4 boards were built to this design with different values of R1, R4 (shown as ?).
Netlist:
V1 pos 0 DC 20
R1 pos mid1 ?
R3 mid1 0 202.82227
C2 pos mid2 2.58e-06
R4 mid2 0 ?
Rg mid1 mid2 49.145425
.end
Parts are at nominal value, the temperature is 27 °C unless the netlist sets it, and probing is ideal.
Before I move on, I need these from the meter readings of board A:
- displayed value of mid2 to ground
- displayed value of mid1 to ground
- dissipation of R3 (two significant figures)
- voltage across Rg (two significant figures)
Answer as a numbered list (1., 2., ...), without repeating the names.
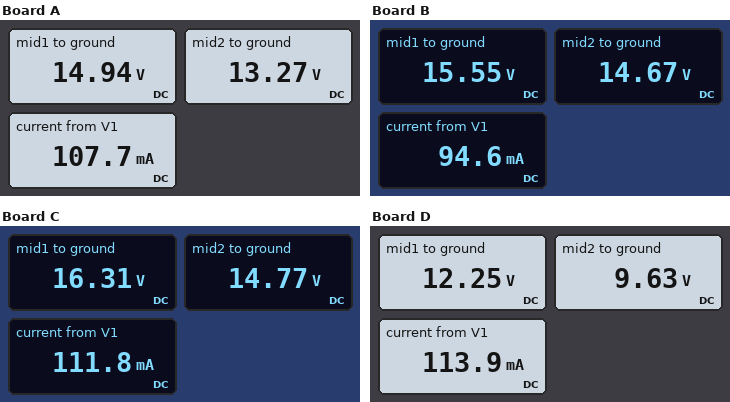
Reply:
1. 13.27 V
2. 14.94 V
3. 1.1 W
4. 1.7 V
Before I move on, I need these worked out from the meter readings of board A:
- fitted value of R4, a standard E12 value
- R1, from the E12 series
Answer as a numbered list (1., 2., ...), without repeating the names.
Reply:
1. 390 Ω
2. 47 Ω
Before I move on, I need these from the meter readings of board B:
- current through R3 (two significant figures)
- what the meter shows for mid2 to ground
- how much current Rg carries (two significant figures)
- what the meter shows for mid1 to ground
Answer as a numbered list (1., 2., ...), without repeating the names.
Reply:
1. 77 mA
2. 14.67 V
3. 18 mA
4. 15.55 V
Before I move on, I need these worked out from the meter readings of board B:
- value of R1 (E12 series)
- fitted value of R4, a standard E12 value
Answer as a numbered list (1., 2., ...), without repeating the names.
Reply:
1. 47 Ω
2. 820 Ω
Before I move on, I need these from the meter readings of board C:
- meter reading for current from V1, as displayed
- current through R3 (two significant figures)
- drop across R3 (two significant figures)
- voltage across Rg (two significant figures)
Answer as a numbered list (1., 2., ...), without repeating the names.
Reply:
1. 111.8 mA
2. 80 mA
3. 16 V
4. 1.5 V
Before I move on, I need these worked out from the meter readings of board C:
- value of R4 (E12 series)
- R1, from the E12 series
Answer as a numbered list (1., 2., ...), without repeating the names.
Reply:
1. 470 Ω
2. 33 Ω
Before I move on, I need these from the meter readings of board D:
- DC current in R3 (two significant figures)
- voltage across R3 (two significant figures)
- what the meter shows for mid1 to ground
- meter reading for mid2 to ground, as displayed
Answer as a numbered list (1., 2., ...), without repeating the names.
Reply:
1. 60 mA
2. 12 V
3. 12.25 V
4. 9.63 V
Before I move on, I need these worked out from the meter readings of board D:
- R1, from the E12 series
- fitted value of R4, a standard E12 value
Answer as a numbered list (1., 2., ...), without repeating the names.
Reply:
1. 68 Ω
2. 180 Ω
